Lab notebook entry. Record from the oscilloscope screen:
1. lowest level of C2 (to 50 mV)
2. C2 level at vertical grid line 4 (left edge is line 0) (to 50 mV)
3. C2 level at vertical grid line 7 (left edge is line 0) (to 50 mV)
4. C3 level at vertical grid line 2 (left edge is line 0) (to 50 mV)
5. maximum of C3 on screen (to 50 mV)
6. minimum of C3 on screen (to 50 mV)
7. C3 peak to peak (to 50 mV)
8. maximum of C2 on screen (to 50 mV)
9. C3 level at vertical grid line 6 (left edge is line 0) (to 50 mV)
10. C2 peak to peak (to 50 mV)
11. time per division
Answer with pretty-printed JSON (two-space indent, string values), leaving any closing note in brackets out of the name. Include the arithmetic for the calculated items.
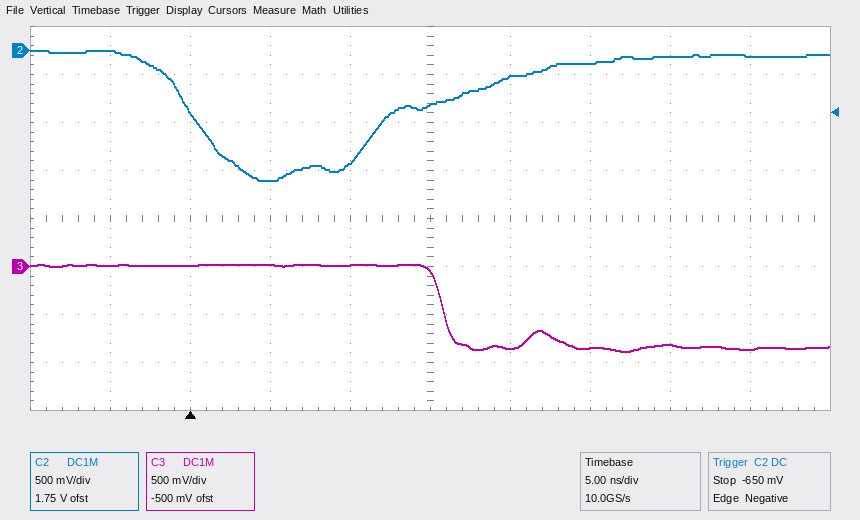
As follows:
{
  "lowest level of C2": "-1.35 V",
  "C2 level at vertical grid line 4 (left edge is line 0)": "-1.15 V",
  "C2 level at vertical grid line 7 (left edge is line 0)": "-150 mV",
  "C3 level at vertical grid line 2 (left edge is line 0)": "0 mV",
  "maximum of C3 on screen": "0 mV",
  "minimum of C3 on screen": "-900 mV",
  "C3 peak to peak": "0 mV − (-900 mV) = 900 mV",
  "maximum of C2 on screen": "0 mV",
  "C3 level at vertical grid line 6 (left edge is line 0)": "-850 mV",
  "C2 peak to peak": "0 mV − (-1.35 V) = 1.35 V",
  "time per division": "5 ns"
}
